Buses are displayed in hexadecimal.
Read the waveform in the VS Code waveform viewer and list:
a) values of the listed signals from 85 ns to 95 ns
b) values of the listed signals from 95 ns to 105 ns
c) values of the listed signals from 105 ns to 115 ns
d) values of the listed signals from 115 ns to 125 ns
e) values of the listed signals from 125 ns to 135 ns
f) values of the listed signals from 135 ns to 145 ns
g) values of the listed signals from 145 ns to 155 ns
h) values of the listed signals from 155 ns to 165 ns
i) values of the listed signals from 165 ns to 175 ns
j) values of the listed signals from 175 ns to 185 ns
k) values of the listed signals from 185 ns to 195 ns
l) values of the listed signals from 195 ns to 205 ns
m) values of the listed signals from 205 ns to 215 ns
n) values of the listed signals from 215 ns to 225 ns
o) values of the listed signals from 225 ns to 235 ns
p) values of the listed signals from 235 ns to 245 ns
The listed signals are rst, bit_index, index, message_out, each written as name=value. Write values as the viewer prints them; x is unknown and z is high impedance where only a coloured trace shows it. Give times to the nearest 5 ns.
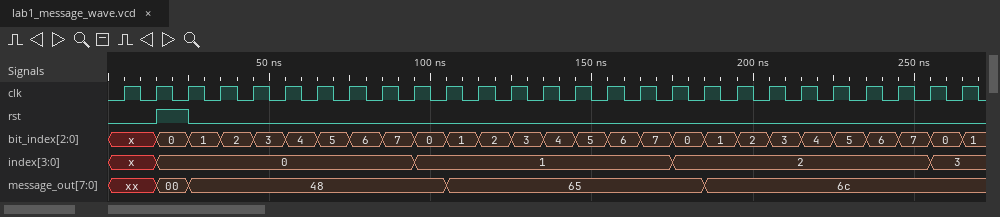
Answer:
rst=0, bit_index=7, index=0, message_out=48
rst=0, bit_index=0, index=1, message_out=48
rst=0, bit_index=1, index=1, message_out=65
rst=0, bit_index=2, index=1, message_out=65
rst=0, bit_index=3, index=1, message_out=65
rst=0, bit_index=4, index=1, message_out=65
rst=0, bit_index=5, index=1, message_out=65
rst=0, bit_index=6, index=1, message_out=65
rst=0, bit_index=7, index=1, message_out=65
rst=0, bit_index=0, index=2, message_out=65
rst=0, bit_index=1, index=2, message_out=6c
rst=0, bit_index=2, index=2, message_out=6c
rst=0, bit_index=3, index=2, message_out=6c
rst=0, bit_index=4, index=2, message_out=6c
rst=0, bit_index=5, index=2, message_out=6c
rst=0, bit_index=6, index=2, message_out=6c
